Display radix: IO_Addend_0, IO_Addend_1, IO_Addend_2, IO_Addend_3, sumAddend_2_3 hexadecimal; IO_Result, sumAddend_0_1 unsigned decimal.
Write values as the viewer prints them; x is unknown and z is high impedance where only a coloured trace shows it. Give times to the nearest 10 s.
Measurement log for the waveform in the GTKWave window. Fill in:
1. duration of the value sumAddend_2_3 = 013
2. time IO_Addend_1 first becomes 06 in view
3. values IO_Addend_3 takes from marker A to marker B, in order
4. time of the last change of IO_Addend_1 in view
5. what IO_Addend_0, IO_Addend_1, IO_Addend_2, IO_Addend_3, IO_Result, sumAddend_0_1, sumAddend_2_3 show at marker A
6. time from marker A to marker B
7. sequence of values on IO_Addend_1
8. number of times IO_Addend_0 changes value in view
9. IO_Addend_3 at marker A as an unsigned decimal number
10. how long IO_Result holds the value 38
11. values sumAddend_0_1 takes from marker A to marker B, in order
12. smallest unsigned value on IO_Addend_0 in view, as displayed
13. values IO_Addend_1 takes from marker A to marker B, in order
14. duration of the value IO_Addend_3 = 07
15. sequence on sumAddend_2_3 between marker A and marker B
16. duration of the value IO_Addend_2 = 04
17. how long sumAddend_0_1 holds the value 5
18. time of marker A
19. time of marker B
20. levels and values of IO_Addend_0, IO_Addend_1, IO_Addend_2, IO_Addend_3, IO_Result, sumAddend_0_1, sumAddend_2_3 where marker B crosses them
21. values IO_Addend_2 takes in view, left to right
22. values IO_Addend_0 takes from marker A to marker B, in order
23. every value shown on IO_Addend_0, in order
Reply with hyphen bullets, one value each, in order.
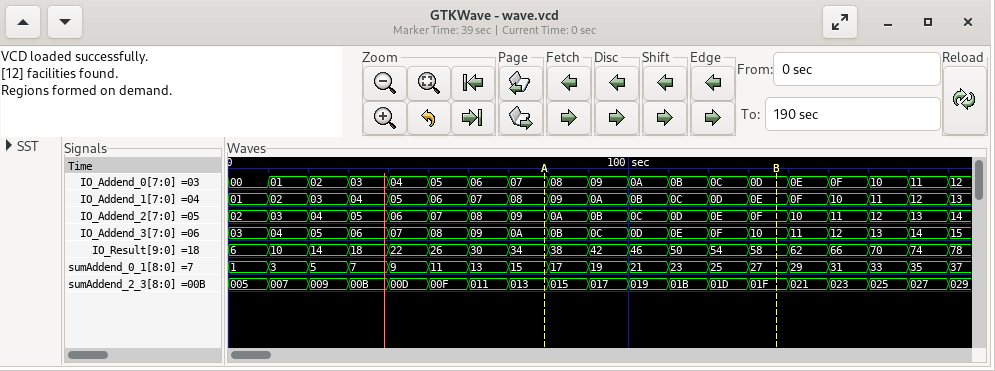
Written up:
- 10 s
- 50 s
- 0A, 0B, 0C, 0D, 0E, 0F, 10
- 180 s
- IO_Addend_0=07, IO_Addend_1=08, IO_Addend_2=09, IO_Addend_3=0A, IO_Result=34, sumAddend_0_1=15, sumAddend_2_3=013
- 60 s
- 01, 02, 03, 04, 05, 06, 07, 08, 09, 0A, 0B, 0C, 0D, 0E, 0F, 10, 11, 12, 13
- 18
- 10
- 10 s
- 15, 17, 19, 21, 23, 25, 27
- 00
- 08, 09, 0A, 0B, 0C, 0D, 0E
- 10 s
- 013, 015, 017, 019, 01B, 01D, 01F
- 10 s
- 10 s
- 80 s
- 140 s
- IO_Addend_0=0D, IO_Addend_1=0E, IO_Addend_2=0F, IO_Addend_3=10, IO_Result=58, sumAddend_0_1=27, sumAddend_2_3=01F
- 02, 03, 04, 05, 06, 07, 08, 09, 0A, 0B, 0C, 0D, 0E, 0F, 10, 11, 12, 13, 14
- 07, 08, 09, 0A, 0B, 0C, 0D
- 00, 01, 02, 03, 04, 05, 06, 07, 08, 09, 0A, 0B, 0C, 0D, 0E, 0F, 10, 11, 12
